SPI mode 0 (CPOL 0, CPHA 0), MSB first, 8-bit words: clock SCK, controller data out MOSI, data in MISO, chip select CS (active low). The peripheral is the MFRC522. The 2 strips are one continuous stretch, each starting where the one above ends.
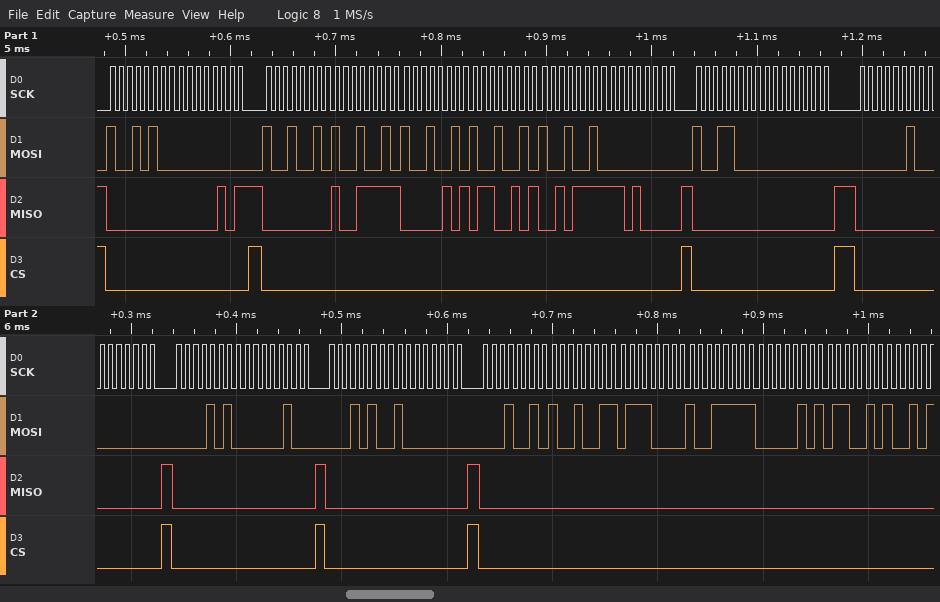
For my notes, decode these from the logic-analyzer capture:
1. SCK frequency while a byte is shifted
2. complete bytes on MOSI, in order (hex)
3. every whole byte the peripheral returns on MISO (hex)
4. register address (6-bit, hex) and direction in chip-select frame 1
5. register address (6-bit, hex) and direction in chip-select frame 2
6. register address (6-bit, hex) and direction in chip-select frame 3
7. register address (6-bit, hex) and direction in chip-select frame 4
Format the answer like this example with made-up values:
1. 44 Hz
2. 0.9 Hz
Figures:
1. 125 kHz
2. 94 00 92 92 92 92 92 00 98 00 02 00 0A 04 14 80 12 93 70 9F 05 65
3. 00 05 00 9F 05 65 2F D0 00 00 00 00 00 00 00 00 00 00 00 00 00 00
4. 0x0A read
5. 0x09 read
6. 0x0C read
7. 0x01 write
